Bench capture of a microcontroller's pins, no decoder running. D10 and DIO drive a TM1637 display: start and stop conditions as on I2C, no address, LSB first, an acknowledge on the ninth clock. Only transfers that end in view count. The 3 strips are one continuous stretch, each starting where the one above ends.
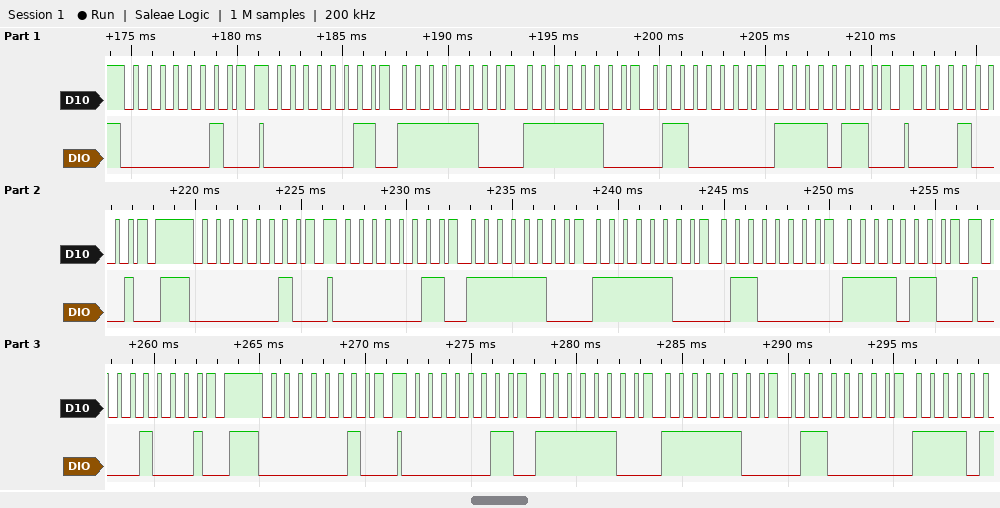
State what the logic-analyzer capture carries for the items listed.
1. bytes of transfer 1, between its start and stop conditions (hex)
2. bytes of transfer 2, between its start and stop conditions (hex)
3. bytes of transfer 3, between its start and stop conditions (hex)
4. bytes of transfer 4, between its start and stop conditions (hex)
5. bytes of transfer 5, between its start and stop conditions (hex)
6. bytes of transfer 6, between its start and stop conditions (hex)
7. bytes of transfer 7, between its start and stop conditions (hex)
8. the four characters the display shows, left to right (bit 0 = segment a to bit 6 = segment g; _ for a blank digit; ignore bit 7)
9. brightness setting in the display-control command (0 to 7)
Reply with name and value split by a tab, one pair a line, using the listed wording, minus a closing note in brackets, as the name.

bytes of transfer 1, between its start and stop conditions	40
bytes of transfer 2, between its start and stop conditions	C0 3F 3F 06 6F
bytes of transfer 3, between its start and stop conditions	88
bytes of transfer 4, between its start and stop conditions	40
bytes of transfer 5, between its start and stop conditions	C0 3F 3F 06 6F
bytes of transfer 6, between its start and stop conditions	88
bytes of transfer 7, between its start and stop conditions	40
the four characters the display shows, left to right	0019
brightness setting in the display-control command	0
